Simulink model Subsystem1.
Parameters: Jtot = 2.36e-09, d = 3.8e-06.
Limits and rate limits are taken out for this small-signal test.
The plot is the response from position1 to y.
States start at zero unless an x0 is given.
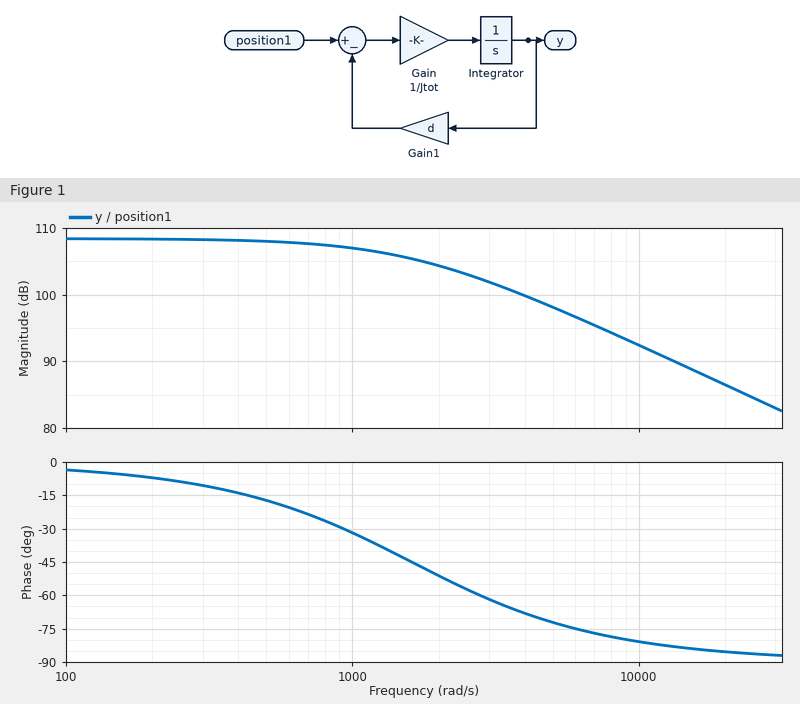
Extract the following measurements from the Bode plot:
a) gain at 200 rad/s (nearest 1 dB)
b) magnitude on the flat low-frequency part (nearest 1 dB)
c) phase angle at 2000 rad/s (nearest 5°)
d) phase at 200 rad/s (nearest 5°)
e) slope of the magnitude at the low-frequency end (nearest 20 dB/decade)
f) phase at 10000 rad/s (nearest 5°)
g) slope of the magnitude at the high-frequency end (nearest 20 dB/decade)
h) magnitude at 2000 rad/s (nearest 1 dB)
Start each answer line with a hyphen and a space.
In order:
- 108 dB
- 108 dB
- -50°
- -5°
- 0 dB/decade
- -80°
- -20 dB/decade
- 104 dB
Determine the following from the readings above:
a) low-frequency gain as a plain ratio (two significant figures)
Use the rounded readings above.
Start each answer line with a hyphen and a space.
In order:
- 250000
